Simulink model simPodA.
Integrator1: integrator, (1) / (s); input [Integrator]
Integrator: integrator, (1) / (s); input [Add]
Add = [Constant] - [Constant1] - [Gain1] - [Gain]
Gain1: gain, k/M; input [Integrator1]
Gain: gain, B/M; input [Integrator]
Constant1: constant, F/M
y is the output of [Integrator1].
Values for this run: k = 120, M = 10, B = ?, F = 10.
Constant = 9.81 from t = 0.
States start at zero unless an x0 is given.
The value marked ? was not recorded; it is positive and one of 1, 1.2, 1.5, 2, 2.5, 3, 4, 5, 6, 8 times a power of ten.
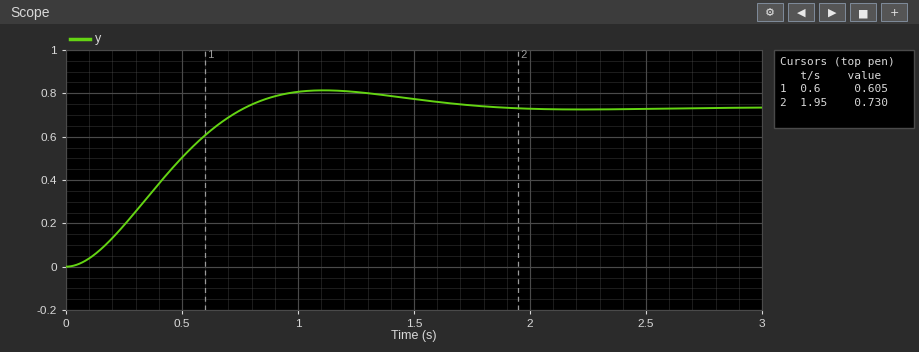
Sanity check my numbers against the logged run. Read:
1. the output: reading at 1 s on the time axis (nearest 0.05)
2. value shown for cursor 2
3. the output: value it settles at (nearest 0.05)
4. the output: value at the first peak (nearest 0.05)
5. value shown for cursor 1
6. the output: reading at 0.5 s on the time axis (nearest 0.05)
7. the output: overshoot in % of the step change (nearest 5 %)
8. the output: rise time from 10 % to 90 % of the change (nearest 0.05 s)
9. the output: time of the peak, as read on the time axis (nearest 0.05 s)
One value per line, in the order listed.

0.80
0.730
0.75
0.80
0.605
0.50
10 %
0.50 s
1.10 s
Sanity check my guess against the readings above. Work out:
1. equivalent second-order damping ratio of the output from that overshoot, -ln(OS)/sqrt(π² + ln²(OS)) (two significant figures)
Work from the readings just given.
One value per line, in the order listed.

0.59
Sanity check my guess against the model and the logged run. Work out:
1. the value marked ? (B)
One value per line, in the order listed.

40
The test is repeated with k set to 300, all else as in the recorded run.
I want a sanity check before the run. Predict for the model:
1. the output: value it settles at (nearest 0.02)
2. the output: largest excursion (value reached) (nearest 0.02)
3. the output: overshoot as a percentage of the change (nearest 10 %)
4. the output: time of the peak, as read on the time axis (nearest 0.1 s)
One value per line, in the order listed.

0.30
0.38
30 %
0.6 s
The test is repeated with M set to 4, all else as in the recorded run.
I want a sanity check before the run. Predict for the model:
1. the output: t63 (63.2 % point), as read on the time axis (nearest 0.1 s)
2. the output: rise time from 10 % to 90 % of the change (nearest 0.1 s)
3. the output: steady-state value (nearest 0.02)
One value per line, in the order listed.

0.4 s
0.5 s
0.24
